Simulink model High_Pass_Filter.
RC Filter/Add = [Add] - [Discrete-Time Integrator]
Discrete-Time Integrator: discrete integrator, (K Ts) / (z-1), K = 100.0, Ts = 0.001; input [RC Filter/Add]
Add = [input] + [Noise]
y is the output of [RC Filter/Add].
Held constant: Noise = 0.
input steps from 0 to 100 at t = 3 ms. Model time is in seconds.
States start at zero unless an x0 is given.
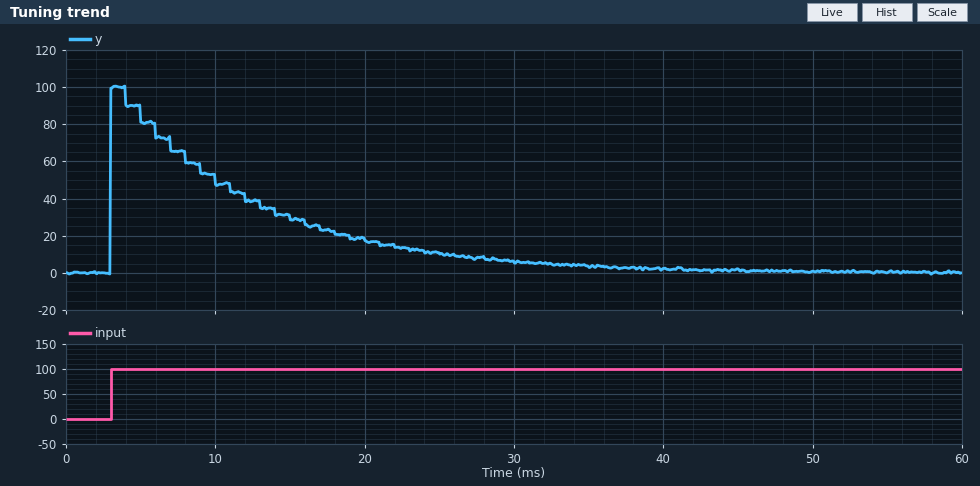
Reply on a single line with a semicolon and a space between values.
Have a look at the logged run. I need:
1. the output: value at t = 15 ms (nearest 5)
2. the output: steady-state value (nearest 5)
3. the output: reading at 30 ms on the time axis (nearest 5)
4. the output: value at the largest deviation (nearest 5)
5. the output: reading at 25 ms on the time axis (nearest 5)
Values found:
30; 0; 5; 100; 10
